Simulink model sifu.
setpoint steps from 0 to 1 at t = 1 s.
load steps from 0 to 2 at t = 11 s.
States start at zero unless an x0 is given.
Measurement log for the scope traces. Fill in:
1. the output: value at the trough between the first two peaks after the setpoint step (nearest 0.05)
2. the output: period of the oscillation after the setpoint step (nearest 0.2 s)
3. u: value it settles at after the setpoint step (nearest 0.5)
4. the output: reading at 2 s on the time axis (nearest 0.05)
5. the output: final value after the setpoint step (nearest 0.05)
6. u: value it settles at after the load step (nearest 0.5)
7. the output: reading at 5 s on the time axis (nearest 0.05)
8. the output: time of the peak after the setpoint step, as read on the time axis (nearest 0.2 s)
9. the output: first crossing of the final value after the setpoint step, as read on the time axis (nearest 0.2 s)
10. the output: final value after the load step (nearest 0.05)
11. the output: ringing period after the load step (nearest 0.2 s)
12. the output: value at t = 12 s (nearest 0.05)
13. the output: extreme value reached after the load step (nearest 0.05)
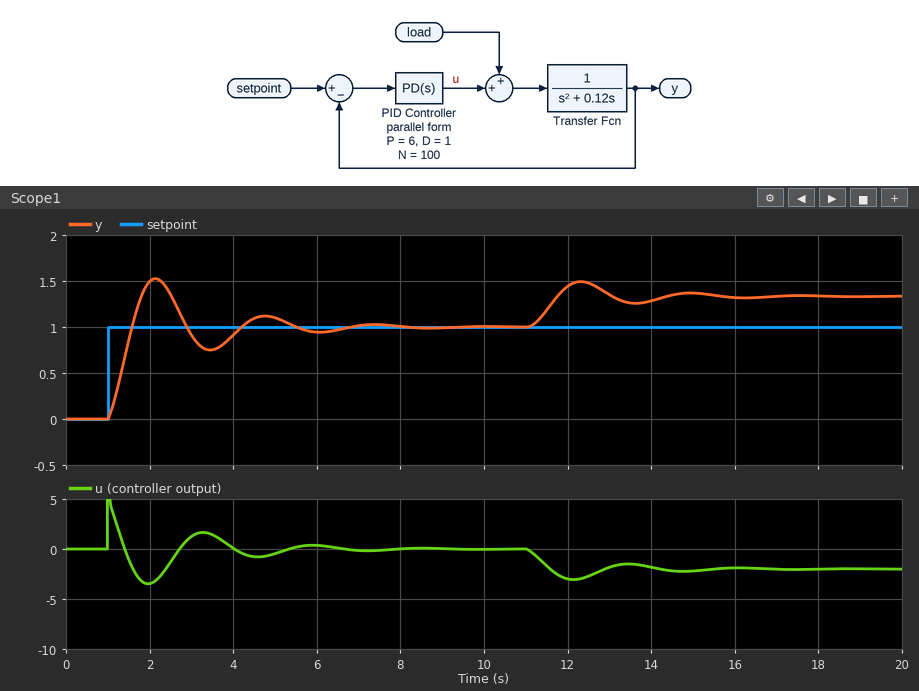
0.75
2.6 s
0.0
1.50
1.00
-2.0
1.10
2.2 s
1.6 s
1.35
2.6 s
1.45
1.50
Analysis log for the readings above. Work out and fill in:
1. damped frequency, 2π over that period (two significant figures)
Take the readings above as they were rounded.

2.4 rad/s
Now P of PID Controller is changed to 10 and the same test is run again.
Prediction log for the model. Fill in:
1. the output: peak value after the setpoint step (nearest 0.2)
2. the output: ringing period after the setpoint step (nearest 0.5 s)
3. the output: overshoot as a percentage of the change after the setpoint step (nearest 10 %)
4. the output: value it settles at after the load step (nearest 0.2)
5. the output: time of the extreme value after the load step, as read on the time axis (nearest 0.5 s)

1.6
2.0 s
60 %
1.2
12.0 s
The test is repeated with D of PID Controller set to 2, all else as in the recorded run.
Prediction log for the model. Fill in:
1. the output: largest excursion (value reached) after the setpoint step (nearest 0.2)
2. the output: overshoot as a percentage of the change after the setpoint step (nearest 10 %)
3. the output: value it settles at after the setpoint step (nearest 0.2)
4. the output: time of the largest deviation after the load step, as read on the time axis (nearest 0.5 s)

1.4
30 %
1.0
12.5 s
